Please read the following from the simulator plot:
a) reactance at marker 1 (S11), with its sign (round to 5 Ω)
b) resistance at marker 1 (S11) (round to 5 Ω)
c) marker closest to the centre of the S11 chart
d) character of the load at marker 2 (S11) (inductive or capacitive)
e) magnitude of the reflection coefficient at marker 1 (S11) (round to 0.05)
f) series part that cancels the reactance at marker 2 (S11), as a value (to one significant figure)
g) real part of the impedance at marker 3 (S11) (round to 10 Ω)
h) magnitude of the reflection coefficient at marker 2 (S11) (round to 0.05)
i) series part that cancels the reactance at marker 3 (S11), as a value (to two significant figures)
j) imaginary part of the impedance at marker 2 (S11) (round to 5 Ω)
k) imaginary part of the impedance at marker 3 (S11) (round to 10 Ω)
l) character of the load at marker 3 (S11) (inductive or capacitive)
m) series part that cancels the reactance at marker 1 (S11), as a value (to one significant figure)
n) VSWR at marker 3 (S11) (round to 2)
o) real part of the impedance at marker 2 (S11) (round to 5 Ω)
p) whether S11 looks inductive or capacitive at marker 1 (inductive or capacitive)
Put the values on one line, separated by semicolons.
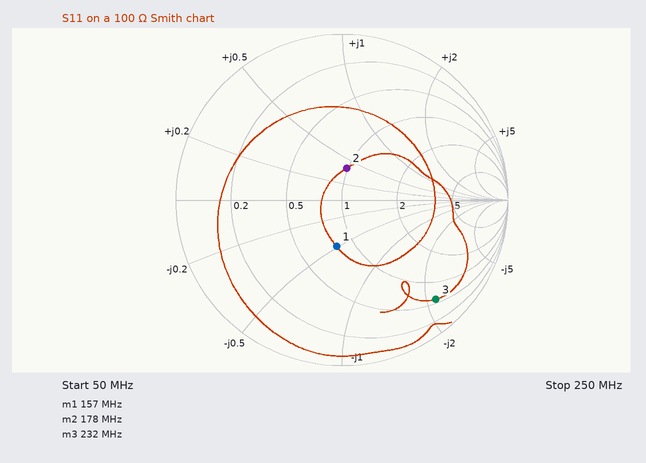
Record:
-50 Ω; 80 Ω; marker 2; inductive; 0.30; 20 pF; 60 Ω; 0.20; 150 nH; +40 Ω; -220 Ω; capacitive; 50 nH; 10; 100 Ω; capacitive
